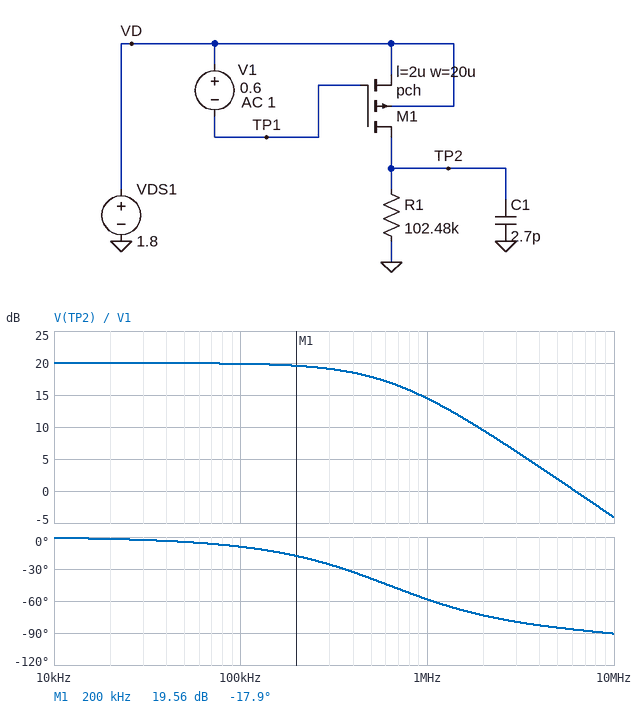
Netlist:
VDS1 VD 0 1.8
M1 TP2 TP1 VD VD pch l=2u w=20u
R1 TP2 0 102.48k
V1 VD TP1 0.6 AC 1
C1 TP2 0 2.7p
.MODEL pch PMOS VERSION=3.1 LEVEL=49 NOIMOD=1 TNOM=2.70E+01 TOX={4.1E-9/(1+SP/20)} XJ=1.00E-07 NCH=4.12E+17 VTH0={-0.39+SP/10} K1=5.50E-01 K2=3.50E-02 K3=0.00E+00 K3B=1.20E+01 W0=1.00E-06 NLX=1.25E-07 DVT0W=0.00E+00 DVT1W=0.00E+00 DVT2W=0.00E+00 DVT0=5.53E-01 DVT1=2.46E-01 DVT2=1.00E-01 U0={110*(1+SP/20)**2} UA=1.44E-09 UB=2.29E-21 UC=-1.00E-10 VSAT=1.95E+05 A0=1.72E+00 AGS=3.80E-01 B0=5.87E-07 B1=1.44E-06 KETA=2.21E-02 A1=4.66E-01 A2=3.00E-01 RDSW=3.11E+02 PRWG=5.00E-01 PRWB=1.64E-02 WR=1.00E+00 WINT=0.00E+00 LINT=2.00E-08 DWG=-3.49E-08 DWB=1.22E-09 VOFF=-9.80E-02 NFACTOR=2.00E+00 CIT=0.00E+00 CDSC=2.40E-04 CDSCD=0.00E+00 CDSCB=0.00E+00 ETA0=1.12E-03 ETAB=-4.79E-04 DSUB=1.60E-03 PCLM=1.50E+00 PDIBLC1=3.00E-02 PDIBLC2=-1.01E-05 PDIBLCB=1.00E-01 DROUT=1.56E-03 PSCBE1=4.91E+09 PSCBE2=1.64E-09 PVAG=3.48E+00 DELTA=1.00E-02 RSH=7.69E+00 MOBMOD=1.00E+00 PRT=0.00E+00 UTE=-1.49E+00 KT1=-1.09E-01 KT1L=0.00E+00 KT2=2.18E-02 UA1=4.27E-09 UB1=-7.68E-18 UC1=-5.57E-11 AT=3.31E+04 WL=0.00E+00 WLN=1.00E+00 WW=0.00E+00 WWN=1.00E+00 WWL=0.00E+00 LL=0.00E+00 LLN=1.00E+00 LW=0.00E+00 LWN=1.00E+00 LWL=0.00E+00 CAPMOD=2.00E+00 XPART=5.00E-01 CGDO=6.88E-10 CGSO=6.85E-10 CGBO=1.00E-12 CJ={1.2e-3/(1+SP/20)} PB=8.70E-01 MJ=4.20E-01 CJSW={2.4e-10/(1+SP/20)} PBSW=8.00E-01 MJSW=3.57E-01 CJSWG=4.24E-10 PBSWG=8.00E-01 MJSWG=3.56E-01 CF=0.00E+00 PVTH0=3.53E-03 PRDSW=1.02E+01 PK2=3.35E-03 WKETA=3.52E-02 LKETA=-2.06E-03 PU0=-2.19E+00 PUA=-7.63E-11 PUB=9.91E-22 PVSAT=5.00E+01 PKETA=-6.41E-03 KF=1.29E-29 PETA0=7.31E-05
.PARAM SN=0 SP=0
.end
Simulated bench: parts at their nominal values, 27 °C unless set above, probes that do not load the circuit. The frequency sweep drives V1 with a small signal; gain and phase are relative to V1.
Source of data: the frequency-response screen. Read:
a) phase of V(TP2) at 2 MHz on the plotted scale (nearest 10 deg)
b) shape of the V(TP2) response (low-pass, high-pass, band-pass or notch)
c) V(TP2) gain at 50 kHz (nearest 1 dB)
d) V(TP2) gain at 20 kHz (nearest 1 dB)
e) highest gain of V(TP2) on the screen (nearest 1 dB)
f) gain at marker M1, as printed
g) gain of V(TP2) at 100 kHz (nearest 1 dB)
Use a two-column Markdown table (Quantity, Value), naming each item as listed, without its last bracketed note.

| Quantity | Value |
|---|---|
| phase of V(TP2) at 2 MHz on the plotted scale | -70 deg |
| shape of the V(TP2) response | low-pass |
| V(TP2) gain at 50 kHz | 20 dB |
| V(TP2) gain at 20 kHz | 20 dB |
| highest gain of V(TP2) on the screen | 20 dB |
| gain at marker M1, as printed | 19.56 dB |
| gain of V(TP2) at 100 kHz | 20 dB |
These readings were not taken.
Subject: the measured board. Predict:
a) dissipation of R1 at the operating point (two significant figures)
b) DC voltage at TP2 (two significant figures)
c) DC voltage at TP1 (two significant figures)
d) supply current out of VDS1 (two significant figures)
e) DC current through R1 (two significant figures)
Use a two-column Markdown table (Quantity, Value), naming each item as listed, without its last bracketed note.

| Quantity | Value |
|---|---|
| dissipation of R1 at the operating point | 13 µW |
| DC voltage at TP2 | 1.1 V |
| DC voltage at TP1 | 1.2 V |
| supply current out of VDS1 | 11 µA |
| DC current through R1 | 11 µA |
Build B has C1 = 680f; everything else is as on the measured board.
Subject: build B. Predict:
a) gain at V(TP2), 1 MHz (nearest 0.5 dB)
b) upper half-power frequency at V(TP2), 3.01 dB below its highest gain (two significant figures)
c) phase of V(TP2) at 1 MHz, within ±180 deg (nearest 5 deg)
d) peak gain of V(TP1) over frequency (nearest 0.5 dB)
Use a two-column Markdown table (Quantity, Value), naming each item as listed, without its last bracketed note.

| Quantity | Value |
|---|---|
| gain at V(TP2), 1 MHz | 19.5 dB |
| upper half-power frequency at V(TP2), 3.01 dB below its highest gain | 2.4 MHz |
| phase of V(TP2) at 1 MHz, within ±180 deg | -25 deg |
| peak gain of V(TP1) over frequency | 0 dB |
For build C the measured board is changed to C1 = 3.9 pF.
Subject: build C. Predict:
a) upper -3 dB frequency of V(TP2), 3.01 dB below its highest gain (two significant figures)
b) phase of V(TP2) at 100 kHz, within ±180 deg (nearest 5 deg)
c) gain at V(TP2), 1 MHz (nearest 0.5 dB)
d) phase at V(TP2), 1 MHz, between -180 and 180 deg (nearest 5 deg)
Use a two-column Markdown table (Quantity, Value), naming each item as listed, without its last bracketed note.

| Quantity | Value |
|---|---|
| upper -3 dB frequency of V(TP2), 3.01 dB below its highest gain | 430 kHz |
| phase of V(TP2) at 100 kHz, within ±180 deg | -15 deg |
| gain at V(TP2), 1 MHz | 12.0 dB |
| phase at V(TP2), 1 MHz, between -180 and 180 deg | -65 deg |
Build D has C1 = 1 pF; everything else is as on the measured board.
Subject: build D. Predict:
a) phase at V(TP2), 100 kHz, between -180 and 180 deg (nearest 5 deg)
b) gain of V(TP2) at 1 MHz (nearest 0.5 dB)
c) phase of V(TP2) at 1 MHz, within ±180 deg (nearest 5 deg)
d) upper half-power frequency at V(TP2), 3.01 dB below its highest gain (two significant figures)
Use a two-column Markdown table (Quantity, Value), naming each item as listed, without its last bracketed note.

| Quantity | Value |
|---|---|
| phase at V(TP2), 100 kHz, between -180 and 180 deg | -5 deg |
| gain of V(TP2) at 1 MHz | 18.5 dB |
| phase of V(TP2) at 1 MHz, within ±180 deg | -30 deg |
| upper half-power frequency at V(TP2), 3.01 dB below its highest gain | 1.7 MHz |
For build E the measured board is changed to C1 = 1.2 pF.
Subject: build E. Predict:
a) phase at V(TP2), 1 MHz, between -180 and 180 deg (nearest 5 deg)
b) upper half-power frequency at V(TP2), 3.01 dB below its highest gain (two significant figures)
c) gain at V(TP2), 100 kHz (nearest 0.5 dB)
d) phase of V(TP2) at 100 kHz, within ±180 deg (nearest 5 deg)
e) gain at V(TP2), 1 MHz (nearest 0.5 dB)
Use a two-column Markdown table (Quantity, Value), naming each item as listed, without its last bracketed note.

| Quantity | Value |
|---|---|
| phase at V(TP2), 1 MHz, between -180 and 180 deg | -35 deg |
| upper half-power frequency at V(TP2), 3.01 dB below its highest gain | 1.4 MHz |
| gain at V(TP2), 100 kHz | 20.0 dB |
| phase of V(TP2) at 100 kHz, within ±180 deg | -5 deg |
| gain at V(TP2), 1 MHz | 18.0 dB |
